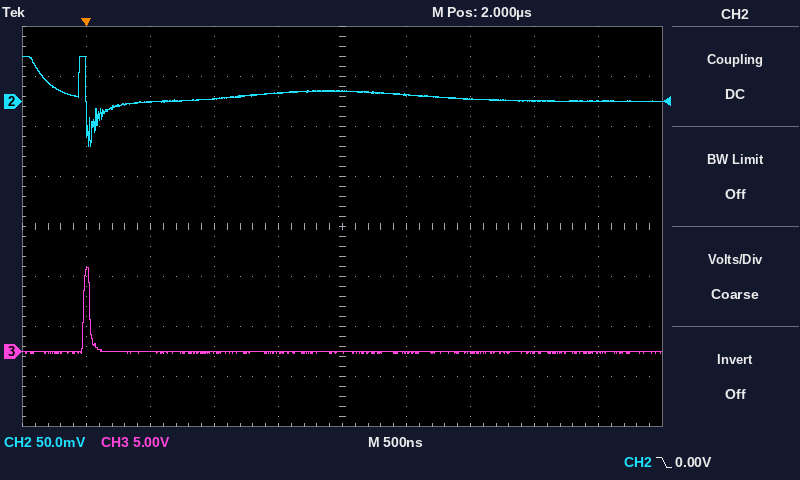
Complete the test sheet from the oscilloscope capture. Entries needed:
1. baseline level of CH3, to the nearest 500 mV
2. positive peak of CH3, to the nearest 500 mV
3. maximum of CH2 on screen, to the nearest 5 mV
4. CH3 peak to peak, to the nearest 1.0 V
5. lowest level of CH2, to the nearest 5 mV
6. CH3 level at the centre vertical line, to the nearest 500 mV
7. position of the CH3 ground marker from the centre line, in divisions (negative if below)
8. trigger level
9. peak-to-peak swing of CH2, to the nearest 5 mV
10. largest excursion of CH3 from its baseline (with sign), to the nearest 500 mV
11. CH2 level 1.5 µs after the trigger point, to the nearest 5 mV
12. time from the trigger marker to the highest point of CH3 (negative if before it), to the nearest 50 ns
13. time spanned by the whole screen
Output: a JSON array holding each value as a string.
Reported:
["0.0 V", "8.5 V", "45 mV", "9.0 V", "-45 mV", "0.0 V", "-2.5 div", "0.00 V", "90 mV", "+8.5 V", "10 mV", "0 ns", "5 µs"]
